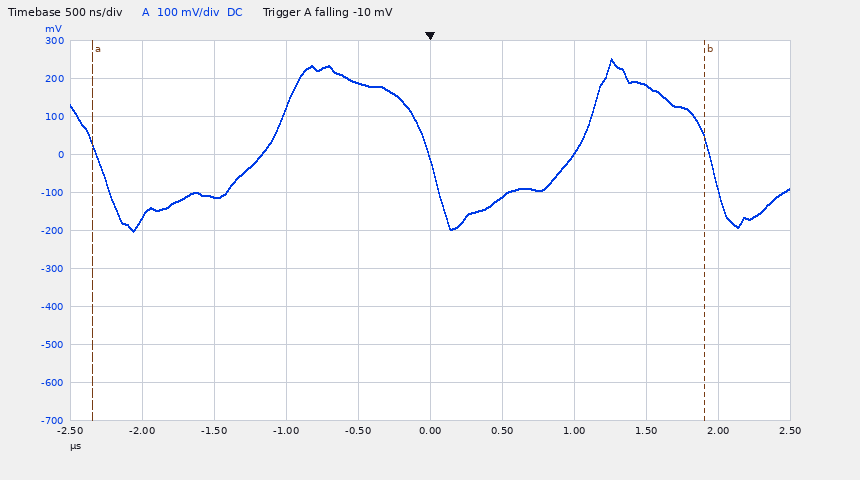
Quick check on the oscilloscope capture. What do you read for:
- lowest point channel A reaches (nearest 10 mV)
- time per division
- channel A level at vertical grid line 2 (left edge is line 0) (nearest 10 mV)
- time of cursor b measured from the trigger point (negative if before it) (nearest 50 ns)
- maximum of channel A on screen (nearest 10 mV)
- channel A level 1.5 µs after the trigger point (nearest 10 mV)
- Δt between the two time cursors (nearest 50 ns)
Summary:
-200 mV
500 ns
-110 mV
+1.90 µs
250 mV
180 mV
4.25 µs
